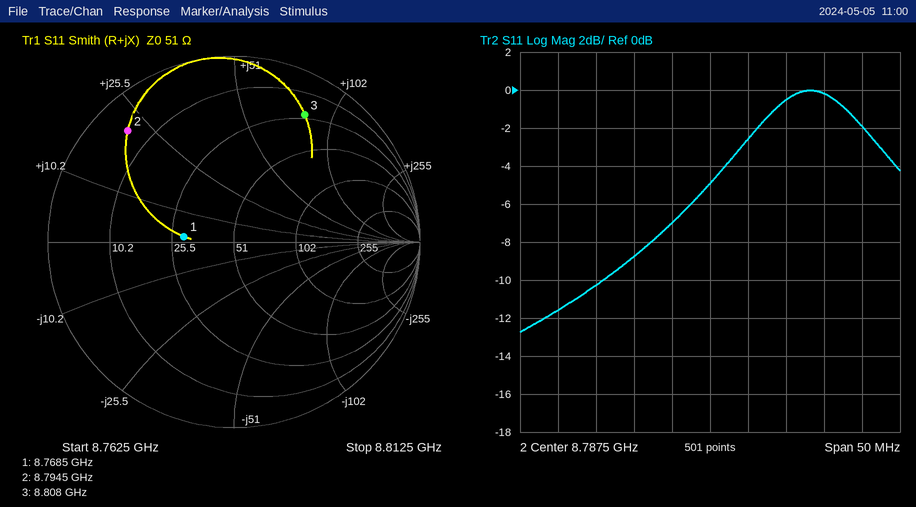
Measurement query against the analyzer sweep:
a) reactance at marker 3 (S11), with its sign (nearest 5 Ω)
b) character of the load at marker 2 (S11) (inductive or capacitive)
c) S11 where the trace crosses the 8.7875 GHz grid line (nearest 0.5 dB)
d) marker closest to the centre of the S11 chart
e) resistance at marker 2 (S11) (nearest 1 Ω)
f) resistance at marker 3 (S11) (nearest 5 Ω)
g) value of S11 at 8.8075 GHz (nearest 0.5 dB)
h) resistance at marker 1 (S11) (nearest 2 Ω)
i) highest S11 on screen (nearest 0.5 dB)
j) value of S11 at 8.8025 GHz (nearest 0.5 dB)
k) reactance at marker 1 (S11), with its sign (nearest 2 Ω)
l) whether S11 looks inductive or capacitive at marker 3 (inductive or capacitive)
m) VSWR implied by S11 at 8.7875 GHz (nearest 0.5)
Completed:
+80 Ω
inductive
-5.0 dB
marker 1
6 Ω
25 Ω
-2.0 dB
30 Ω
0.0 dB
0.0 dB
+2 Ω
inductive
3.5
